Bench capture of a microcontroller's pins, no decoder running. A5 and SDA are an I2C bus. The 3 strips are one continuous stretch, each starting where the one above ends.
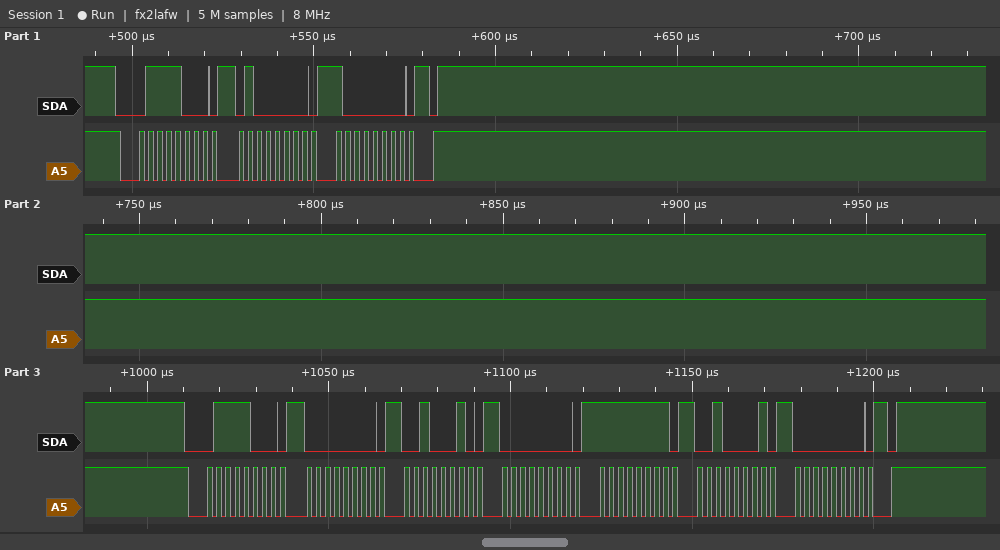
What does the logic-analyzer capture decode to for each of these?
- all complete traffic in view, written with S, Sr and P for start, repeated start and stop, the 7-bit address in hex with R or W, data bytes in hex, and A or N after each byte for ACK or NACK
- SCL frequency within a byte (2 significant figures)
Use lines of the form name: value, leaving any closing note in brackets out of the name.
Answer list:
all complete traffic in view, written with S, Sr and P for start, repeated start and stop, the 7-bit address in hex with R or W, data bytes in hex, and A or N after each byte for ACK or NACK: S 3CW A 40 A 80 A P S 3CW A 00 A 22 A 00 A FF A 21 A 00 A P
SCL frequency within a byte: 400 kHz
